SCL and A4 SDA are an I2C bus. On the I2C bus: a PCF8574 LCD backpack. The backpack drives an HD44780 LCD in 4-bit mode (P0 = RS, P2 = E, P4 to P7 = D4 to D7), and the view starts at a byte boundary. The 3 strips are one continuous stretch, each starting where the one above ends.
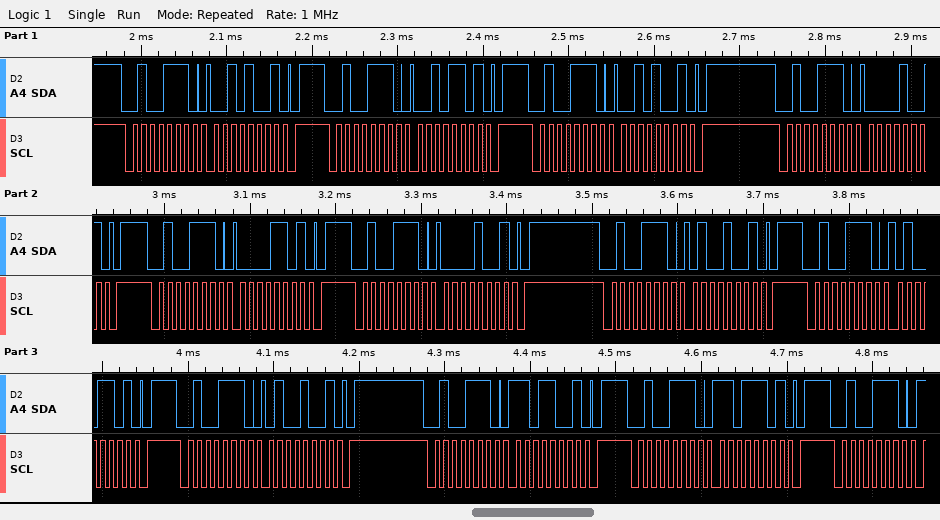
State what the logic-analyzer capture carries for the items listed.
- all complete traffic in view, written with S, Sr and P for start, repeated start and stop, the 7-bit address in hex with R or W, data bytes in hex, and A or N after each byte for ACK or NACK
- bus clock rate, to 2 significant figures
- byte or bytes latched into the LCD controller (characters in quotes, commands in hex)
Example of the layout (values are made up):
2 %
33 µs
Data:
S 27W A 29 A P S 27W A 2D A P S 27W A 29 A P S 27W A 09 A P S 27W A 0D A P S 27W A 09 A P S 27W A 49 A P S 27W A 4D A P S 27W A 49 A P S 27W A D9 A P S 27W A DD A P S 27W A
100 kHz
' '
